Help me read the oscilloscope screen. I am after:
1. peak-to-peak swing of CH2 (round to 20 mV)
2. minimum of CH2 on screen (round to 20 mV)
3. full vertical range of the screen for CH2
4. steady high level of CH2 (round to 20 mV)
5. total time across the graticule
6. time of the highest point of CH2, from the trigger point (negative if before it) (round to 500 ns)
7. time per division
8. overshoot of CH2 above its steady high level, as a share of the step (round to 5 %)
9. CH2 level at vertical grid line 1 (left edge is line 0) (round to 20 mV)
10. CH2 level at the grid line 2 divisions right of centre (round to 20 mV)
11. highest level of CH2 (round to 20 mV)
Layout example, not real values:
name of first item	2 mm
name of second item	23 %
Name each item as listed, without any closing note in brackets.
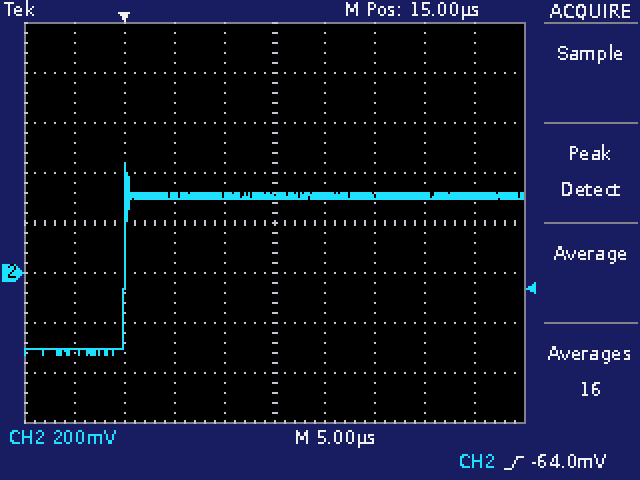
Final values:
peak-to-peak swing of CH2	760 mV
minimum of CH2 on screen	-320 mV
full vertical range of the screen for CH2	1.6 V
steady high level of CH2	300 mV
total time across the graticule	50 µs
time of the highest point of CH2, from the trigger point (negative if before it)	0.0 µs
time per division	5 µs
overshoot of CH2 above its steady high level, as a share of the step	20 %
CH2 level at vertical grid line 1 (left edge is line 0)	-300 mV
CH2 level at the grid line 2 divisions right of centre	300 mV
highest level of CH2	440 mV
